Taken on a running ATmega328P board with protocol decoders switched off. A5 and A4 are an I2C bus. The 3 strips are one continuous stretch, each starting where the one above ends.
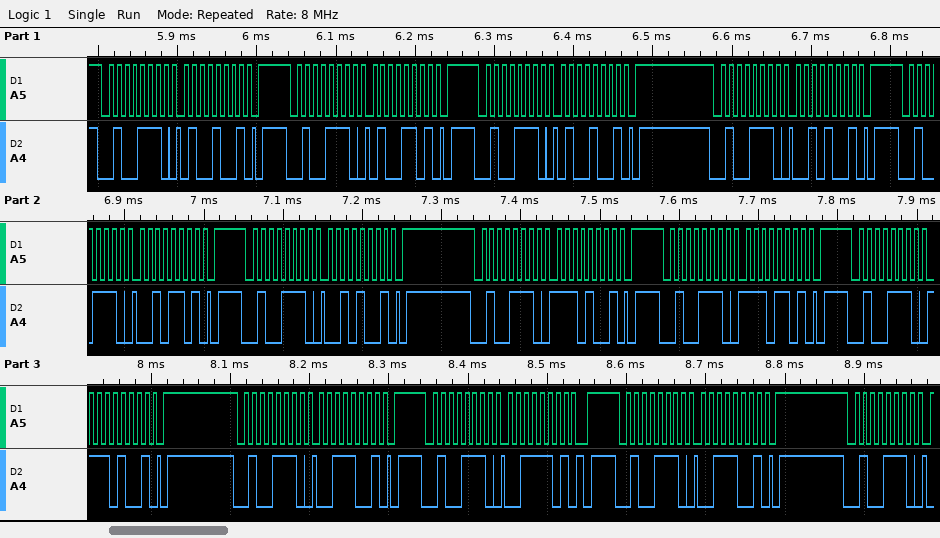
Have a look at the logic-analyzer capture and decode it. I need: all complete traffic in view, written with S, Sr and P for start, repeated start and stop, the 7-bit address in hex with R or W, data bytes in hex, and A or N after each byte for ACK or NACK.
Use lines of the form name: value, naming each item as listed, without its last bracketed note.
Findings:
all complete traffic in view, written with S, Sr and P for start, repeated start and stop, the 7-bit address in hex with R or W, data bytes in hex, and A or N after each byte for ACK or NACK: S 27W A 49 A P S 27W A 4D A P S 27W A 49 A P S 27W A 29 A P S 27W A 2D A P S 27W A 29 A P S 27W A E9 A P S 27W A ED A P S 27W A E9 A P S 27W A 39 A P S 27W A 3D A P S 27W A 39 A P S 27W A
